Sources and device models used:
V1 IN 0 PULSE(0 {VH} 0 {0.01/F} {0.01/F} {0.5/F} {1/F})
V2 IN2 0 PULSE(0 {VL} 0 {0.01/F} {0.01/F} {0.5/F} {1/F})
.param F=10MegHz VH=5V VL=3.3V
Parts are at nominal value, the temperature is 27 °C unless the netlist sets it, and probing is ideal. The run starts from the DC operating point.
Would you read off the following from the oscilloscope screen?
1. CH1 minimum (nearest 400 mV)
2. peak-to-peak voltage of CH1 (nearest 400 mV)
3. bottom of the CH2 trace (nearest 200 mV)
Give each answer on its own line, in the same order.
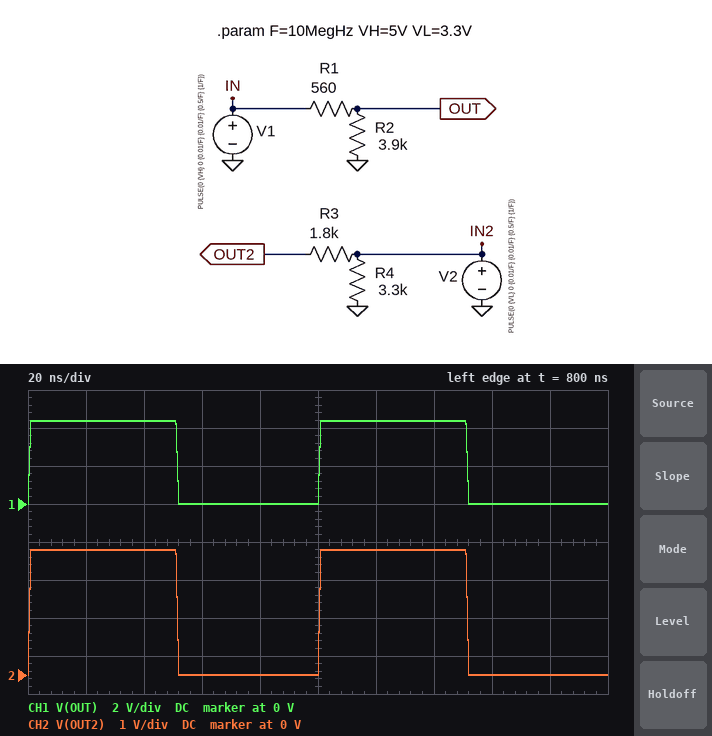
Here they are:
0 V
4.4 V
0 V
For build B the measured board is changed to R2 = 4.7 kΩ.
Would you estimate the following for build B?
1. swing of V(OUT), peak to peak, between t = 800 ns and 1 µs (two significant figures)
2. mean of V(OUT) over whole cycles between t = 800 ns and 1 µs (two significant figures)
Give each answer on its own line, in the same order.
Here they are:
4.5 V
2.3 V
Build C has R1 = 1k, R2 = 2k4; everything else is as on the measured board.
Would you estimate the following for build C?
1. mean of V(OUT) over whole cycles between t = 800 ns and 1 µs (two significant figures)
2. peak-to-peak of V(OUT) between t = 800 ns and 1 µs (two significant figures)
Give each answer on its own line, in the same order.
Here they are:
1.8 V
3.5 V
